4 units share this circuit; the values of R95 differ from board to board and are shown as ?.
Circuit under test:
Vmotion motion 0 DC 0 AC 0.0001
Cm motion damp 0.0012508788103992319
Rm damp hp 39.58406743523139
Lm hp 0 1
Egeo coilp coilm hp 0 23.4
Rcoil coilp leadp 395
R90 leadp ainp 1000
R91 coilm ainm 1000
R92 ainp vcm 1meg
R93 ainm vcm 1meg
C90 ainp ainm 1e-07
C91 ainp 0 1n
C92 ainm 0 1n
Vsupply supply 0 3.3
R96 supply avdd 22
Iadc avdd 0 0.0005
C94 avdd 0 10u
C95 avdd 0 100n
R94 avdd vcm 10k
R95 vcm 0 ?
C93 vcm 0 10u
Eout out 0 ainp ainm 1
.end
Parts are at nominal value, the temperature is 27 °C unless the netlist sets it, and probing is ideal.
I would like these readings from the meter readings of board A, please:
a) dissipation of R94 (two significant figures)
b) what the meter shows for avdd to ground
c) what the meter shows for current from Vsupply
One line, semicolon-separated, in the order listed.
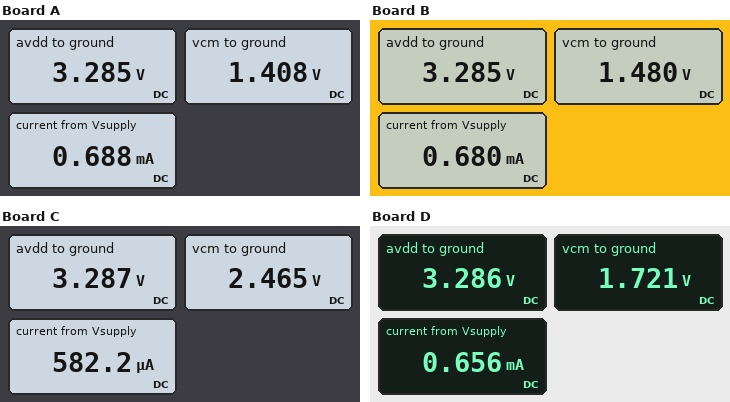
350 µW; 3.285 V; 0.688 mA
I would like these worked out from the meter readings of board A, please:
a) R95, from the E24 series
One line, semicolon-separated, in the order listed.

7.5 kΩ
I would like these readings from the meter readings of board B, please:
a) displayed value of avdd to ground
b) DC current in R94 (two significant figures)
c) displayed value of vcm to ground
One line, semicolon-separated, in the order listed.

3.285 V; 180 µA; 1.480 V
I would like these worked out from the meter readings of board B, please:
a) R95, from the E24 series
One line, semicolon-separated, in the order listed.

8.2 kΩ
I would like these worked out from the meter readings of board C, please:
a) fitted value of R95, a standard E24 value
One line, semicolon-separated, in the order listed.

30 kΩ
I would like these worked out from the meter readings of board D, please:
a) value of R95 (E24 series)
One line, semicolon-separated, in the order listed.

11 kΩ
